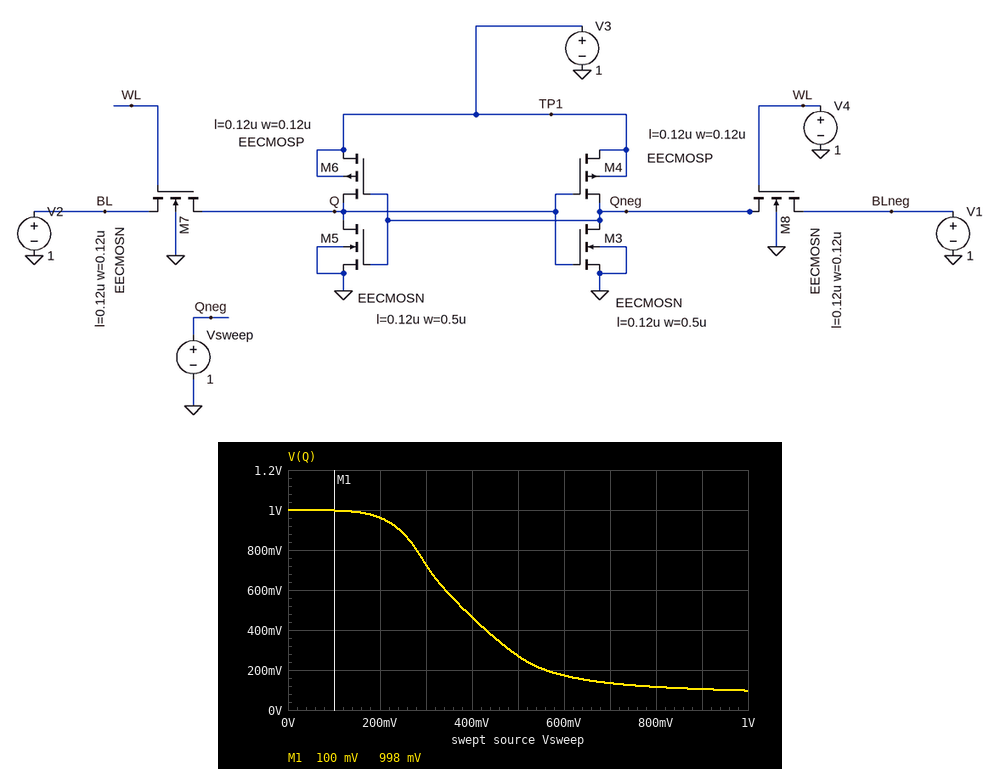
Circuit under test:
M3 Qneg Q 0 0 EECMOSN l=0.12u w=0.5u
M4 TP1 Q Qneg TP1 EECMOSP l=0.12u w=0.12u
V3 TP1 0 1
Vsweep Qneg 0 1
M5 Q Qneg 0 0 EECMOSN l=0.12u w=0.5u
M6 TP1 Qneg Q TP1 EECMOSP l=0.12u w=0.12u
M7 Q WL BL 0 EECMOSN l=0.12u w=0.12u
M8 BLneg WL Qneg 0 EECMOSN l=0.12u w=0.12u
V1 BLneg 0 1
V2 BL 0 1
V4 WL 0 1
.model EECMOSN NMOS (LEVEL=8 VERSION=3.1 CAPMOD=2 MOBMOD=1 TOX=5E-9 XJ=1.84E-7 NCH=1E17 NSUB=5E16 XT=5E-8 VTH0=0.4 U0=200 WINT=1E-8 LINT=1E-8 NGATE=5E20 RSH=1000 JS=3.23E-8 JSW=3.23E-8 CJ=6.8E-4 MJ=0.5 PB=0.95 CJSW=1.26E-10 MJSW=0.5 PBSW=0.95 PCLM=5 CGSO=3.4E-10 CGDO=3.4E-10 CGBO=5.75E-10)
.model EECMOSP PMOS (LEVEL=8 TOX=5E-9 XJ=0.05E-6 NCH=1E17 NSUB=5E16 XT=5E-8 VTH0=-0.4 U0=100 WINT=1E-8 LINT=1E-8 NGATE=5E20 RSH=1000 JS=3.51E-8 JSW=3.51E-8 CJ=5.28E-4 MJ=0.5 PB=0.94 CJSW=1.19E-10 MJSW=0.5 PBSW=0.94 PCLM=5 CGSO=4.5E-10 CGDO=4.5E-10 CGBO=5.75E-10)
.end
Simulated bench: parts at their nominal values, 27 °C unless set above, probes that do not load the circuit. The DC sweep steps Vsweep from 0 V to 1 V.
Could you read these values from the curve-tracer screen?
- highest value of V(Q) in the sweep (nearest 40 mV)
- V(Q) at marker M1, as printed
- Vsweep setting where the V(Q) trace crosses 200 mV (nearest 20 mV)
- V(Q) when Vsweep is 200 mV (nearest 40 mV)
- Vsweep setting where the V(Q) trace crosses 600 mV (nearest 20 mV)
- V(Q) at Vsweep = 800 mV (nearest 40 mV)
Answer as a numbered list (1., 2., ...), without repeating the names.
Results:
1. 1.00 V
2. 998 mV
3. 560 mV
4. 960 mV
5. 340 mV
6. 120 mV
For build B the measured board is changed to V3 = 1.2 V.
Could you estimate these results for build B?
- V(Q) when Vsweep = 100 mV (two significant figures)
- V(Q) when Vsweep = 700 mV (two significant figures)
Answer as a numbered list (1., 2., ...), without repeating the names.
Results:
1. 1.2 V
2. 150 mV
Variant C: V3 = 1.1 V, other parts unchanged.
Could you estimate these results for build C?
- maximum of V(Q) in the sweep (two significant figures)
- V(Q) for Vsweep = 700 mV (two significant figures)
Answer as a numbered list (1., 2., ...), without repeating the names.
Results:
1. 1.1 V
2. 140 mV
